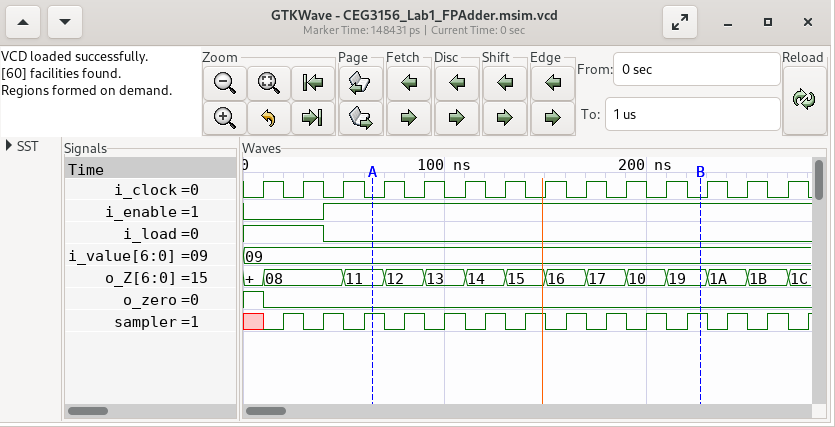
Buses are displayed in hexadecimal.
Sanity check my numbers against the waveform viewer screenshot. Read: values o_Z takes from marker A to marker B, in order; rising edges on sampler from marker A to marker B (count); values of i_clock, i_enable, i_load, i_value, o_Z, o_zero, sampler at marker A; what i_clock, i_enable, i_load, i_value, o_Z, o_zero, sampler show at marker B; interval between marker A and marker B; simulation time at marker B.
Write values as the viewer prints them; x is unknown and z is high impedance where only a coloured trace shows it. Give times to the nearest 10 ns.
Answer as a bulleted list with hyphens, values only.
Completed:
- 11, 12, 13, 14, 15, 16, 17, 10, 19
- 8
- i_clock=0, i_enable=1, i_load=0, i_value=09, o_Z=11, o_zero=0, sampler=1
- i_clock=0, i_enable=1, i_load=0, i_value=09, o_Z=19, o_zero=0, sampler=1
- 160 ns
- 230 ns
